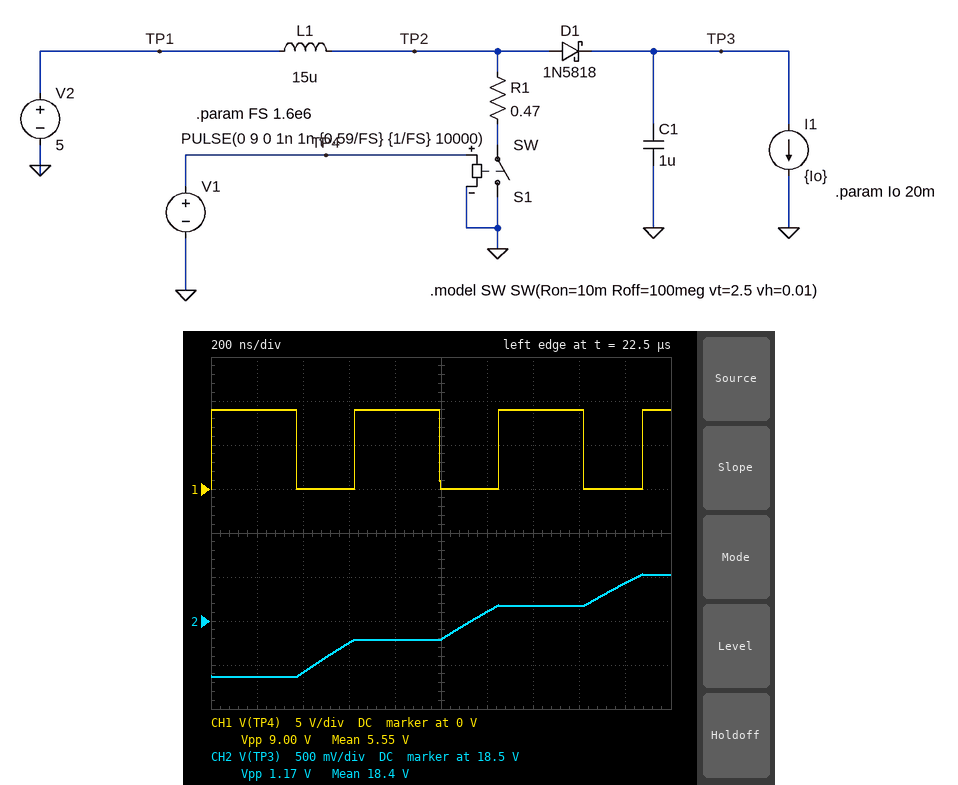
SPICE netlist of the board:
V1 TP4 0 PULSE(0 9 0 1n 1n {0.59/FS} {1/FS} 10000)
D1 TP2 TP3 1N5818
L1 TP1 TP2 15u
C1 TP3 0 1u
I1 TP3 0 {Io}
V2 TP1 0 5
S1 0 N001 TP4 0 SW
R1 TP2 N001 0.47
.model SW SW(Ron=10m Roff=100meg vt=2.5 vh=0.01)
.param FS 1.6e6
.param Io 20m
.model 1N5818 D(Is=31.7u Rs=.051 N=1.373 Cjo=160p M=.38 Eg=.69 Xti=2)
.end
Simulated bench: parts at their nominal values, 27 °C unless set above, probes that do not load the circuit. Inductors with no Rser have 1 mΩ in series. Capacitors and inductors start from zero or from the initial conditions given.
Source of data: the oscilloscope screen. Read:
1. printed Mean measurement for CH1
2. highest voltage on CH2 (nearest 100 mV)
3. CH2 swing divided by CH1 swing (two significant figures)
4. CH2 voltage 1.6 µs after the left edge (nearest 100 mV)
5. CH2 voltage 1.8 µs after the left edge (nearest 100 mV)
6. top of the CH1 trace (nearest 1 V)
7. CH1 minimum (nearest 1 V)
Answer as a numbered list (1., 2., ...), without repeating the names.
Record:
1. 5.55 V
2. 19.0 V
3. 0.13
4. 18.7 V
5. 18.9 V
6. 9 V
7. 0 V
